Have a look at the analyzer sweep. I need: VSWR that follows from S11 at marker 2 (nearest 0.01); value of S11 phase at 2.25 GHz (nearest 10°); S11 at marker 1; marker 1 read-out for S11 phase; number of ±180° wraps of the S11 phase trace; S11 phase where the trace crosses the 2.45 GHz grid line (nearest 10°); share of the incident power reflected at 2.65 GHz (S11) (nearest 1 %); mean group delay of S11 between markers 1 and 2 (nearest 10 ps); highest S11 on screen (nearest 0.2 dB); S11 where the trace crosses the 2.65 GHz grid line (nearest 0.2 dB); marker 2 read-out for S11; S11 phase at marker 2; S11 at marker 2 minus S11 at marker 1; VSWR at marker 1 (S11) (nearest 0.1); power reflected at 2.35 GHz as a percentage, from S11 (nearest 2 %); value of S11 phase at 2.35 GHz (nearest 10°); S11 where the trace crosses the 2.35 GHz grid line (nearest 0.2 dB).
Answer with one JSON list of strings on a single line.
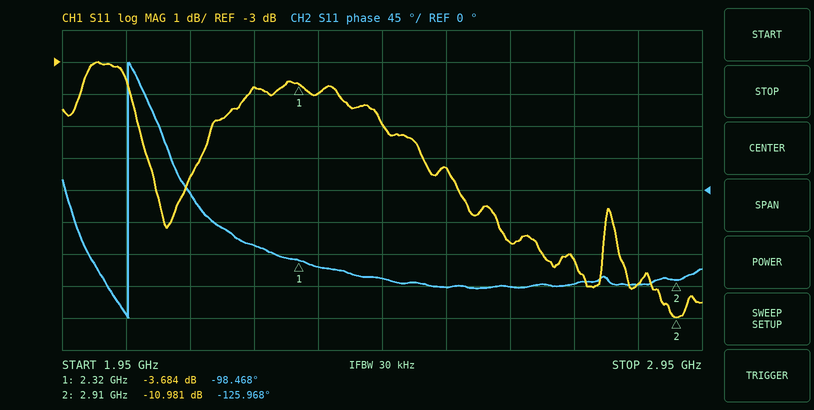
["1.79", "-80°", "-3.684 dB", "-98.468°", "1", "-120°", "14 %", "130 ps", "-3.0 dB", "-8.6 dB", "-10.981 dB", "-125.968°", "-7.297 dB", "4.8", "40 %", "-110°", "-4.0 dB"]
